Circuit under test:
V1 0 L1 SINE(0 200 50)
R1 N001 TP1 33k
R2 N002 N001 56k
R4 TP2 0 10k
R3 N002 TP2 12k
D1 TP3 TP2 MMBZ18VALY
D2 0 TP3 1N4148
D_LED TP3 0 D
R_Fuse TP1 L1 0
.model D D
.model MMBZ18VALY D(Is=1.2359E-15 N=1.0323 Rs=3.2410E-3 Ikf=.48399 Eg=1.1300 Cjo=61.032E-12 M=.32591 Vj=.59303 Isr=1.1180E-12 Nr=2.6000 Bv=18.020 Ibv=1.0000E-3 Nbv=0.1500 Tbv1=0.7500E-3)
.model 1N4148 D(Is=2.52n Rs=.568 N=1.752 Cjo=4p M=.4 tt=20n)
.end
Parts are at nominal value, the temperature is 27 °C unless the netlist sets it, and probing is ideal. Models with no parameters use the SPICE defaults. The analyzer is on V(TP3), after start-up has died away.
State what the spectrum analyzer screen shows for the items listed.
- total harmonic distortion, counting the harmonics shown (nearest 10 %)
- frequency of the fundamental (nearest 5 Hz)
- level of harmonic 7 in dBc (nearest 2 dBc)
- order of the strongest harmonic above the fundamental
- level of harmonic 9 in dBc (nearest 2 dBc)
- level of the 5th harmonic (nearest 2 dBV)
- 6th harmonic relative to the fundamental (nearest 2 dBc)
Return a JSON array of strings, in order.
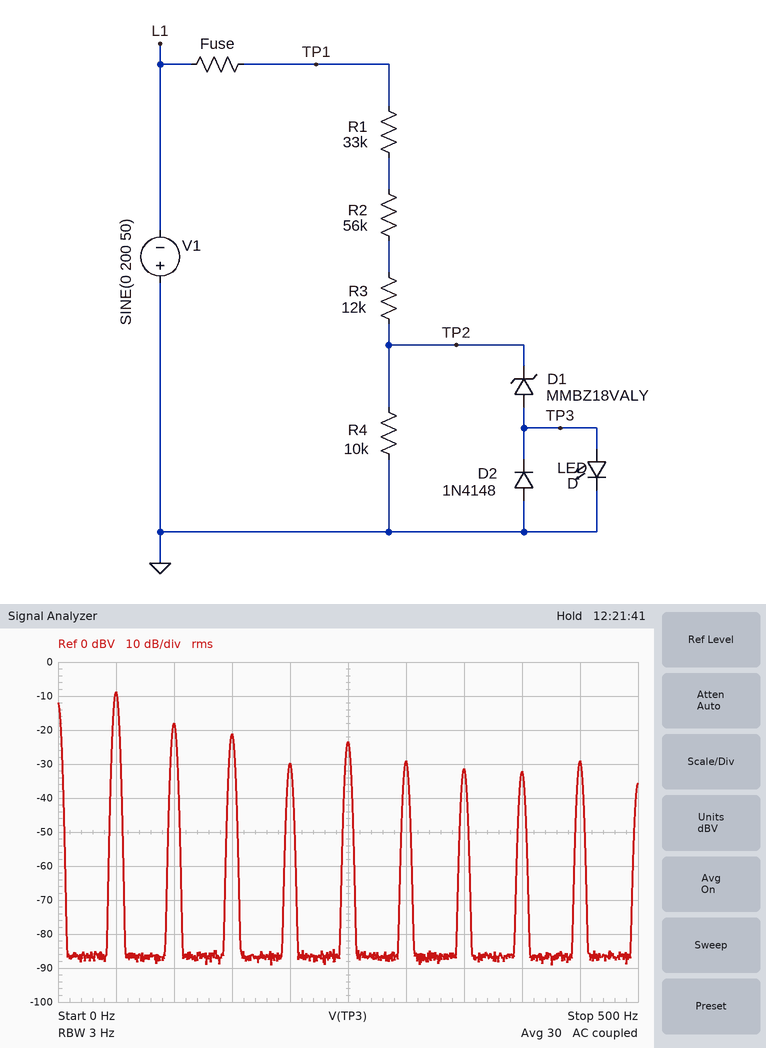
["50 %", "50 Hz", "-22 dBc", "2", "-20 dBc", "-24 dBV", "-20 dBc"]
